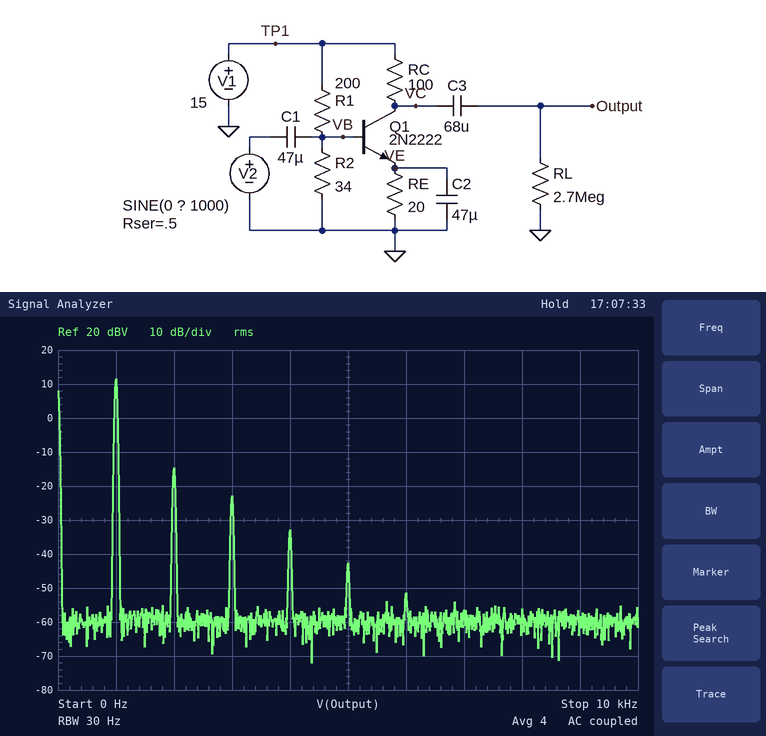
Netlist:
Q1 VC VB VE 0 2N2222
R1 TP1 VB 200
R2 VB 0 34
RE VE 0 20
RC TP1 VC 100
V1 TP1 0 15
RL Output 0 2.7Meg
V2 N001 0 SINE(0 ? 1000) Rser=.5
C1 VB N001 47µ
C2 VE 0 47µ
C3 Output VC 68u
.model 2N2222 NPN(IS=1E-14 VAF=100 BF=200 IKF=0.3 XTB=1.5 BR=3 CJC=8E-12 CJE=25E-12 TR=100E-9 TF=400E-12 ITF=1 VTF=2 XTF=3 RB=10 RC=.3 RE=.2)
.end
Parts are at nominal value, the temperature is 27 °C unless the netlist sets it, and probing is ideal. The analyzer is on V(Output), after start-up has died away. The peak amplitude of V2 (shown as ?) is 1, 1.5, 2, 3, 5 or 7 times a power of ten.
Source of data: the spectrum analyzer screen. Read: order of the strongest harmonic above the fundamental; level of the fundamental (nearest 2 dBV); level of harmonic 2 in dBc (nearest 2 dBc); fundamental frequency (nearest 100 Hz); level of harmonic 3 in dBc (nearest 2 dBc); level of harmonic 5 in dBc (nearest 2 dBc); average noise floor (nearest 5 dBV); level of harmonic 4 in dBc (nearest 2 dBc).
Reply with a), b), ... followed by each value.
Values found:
a) 2
b) 12 dBV
c) -26 dBc
d) 1.0 kHz
e) -34 dBc
f) -54 dBc
g) -60 dBV
h) -44 dBc
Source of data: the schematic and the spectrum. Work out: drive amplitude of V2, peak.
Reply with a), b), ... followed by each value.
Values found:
a) 200 mV
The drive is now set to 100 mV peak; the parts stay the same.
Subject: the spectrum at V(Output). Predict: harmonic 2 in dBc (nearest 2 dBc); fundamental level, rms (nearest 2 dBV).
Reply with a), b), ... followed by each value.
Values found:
a) -34 dBc
b) 6 dBV
